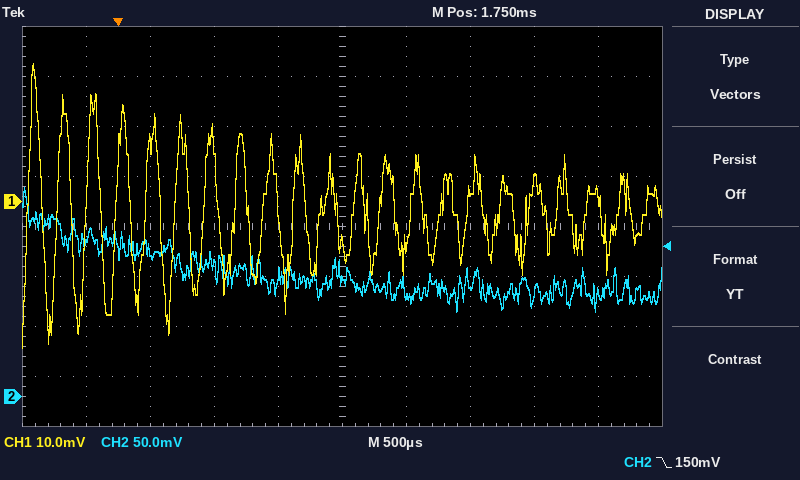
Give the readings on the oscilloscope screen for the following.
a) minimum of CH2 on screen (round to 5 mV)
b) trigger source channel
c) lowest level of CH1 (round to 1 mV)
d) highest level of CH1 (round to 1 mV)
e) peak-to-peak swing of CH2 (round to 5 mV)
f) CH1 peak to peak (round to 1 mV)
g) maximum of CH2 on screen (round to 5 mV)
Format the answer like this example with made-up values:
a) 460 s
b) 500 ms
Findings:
a) 85 mV
b) CH2
c) -29 mV
d) 28 mV
e) 125 mV
f) 57 mV
g) 210 mV
